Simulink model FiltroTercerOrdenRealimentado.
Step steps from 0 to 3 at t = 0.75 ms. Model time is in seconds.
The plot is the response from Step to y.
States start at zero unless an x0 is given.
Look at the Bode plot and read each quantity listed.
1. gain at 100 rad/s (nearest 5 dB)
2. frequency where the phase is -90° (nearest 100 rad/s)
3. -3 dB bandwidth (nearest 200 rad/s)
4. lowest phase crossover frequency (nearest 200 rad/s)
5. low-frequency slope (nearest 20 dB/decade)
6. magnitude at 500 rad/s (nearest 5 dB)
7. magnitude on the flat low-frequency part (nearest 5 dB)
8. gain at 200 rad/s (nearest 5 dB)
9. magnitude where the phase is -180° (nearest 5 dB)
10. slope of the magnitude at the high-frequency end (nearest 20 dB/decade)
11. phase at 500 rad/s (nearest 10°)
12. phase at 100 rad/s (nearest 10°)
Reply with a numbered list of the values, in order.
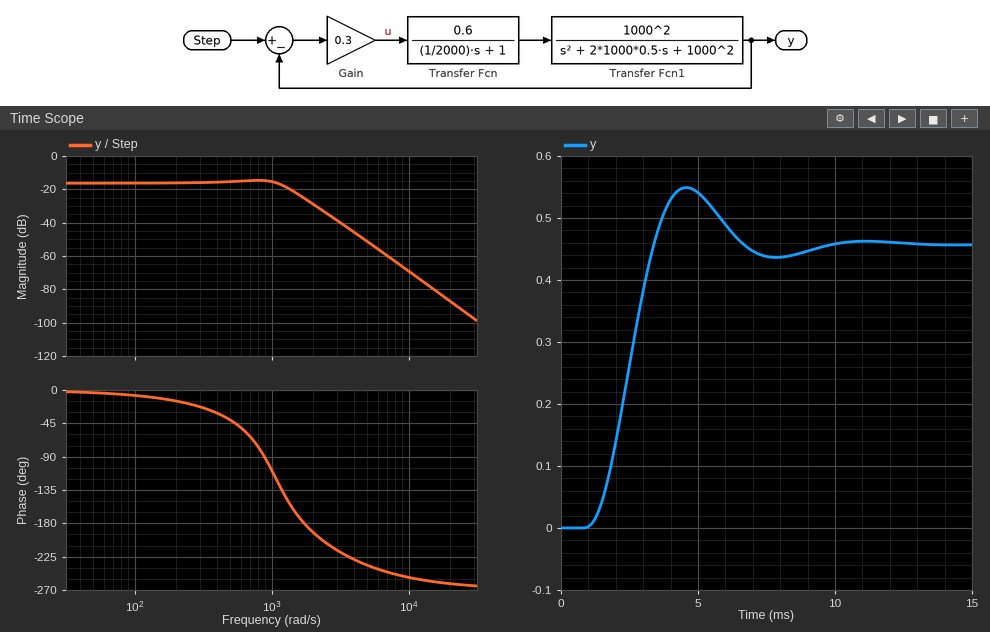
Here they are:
1. -15 dB
2. 900 rad/s
3. 1400 rad/s
4. 1800 rad/s
5. 0 dB/decade
6. -15 dB
7. -15 dB
8. -15 dB
9. -25 dB
10. -60 dB/decade
11. -40°
12. -10°
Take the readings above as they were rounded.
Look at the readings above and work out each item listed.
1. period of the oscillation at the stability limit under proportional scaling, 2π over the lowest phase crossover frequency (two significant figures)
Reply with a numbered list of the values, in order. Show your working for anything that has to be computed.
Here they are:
1. 2π / 1800 = 0.0035 s
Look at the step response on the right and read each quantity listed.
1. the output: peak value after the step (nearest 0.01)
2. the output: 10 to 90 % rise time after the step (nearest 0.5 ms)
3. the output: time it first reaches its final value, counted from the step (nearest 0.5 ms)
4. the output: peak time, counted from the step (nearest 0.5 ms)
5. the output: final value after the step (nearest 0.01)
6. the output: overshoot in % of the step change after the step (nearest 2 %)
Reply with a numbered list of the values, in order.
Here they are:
1. 0.55
2. 1.5 ms
3. 2.5 ms
4. 4.0 ms
5. 0.46
6. 20 %
